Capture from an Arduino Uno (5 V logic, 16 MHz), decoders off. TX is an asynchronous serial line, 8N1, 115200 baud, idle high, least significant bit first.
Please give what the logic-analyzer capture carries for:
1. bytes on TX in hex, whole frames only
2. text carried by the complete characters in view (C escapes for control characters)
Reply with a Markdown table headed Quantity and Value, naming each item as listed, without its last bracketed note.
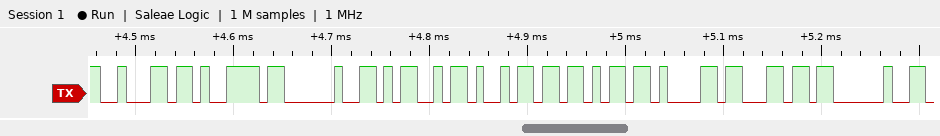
| Quantity | Value |
|---|---|
| bytes on TX in hex, whole frames only | 0x62 0x79 0x20 0x4D 0x69 0x6B 0x61 0x6C 0x20 |
| text carried by the complete characters in view | "by Mikal " |
